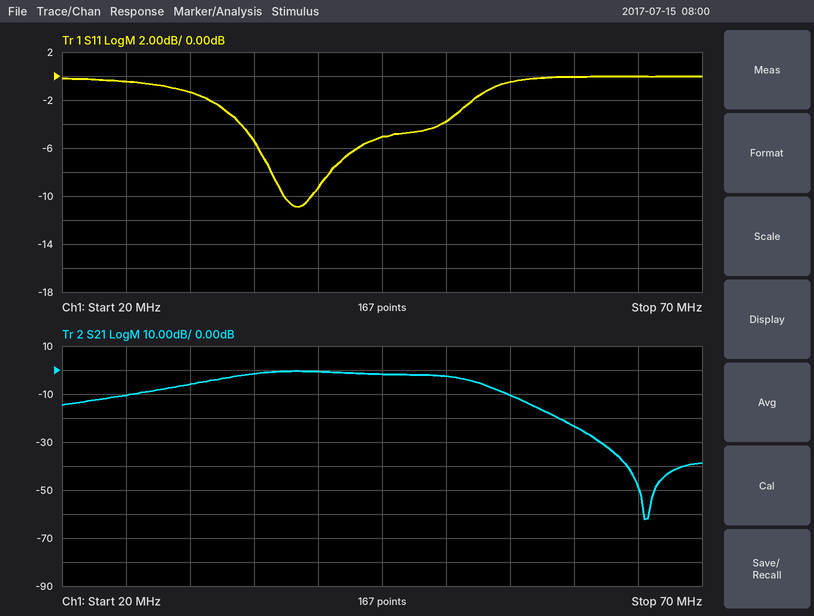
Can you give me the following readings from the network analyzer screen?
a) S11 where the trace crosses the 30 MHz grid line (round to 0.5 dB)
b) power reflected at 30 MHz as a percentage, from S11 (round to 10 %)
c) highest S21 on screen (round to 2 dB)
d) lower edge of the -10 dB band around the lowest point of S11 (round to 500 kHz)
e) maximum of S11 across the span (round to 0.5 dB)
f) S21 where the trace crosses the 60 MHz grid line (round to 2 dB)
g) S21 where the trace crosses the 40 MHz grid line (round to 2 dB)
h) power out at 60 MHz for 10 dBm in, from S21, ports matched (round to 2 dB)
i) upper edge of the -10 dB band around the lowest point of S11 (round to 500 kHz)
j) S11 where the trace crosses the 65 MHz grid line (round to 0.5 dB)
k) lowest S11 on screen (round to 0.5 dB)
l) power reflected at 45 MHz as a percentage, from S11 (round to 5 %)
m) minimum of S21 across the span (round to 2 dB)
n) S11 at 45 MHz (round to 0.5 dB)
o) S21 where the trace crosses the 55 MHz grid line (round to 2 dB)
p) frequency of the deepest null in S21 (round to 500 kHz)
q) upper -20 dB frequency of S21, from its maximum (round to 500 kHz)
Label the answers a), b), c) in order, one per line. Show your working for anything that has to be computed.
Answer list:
a) -1.5 dB
b) 10^(-1.5/10) ≈ 70.8 %, so 70 % to the nearest 10 %
c) 0 dB
d) 37.5 MHz
e) 0.0 dB
f) -24 dB
g) 0 dB
h) 10 dBm + (-24 dB) = -14 dBm
i) 39.5 MHz
j) 0.0 dB
k) -11.0 dB
l) 10^(-5/10) ≈ 31.6 %, so 30 % to the nearest 5 %
m) -62 dB
n) -5.0 dB
o) -10 dB
p) 65.5 MHz
q) 59.0 MHz
